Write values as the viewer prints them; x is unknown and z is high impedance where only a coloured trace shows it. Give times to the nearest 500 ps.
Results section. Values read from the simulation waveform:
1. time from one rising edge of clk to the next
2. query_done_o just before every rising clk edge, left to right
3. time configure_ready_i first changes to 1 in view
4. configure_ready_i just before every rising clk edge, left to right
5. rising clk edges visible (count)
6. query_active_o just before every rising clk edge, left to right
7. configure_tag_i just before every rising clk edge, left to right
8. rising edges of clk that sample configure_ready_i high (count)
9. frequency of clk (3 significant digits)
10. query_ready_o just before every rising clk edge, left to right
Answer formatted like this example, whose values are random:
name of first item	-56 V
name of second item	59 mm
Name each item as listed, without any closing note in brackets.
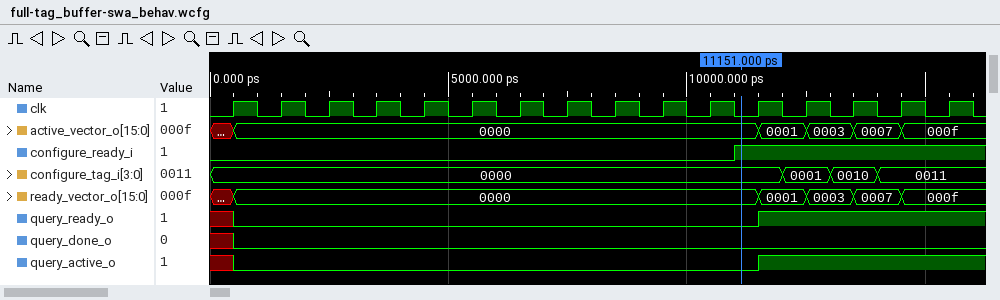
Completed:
time from one rising edge of clk to the next	1000 ps
query_done_o just before every rising clk edge, left to right	x 0 0 0 0 0 0 0 0 0 0 0 0 0 0 0
time configure_ready_i first changes to 1 in view	11000 ps
configure_ready_i just before every rising clk edge, left to right	0 0 0 0 0 0 0 0 0 0 0 1 1 1 1 1
rising clk edges visible	16
query_active_o just before every rising clk edge, left to right	x 0 0 0 0 0 0 0 0 0 0 0 1 1 1 1
configure_tag_i just before every rising clk edge, left to right	0000, 0000, 0000, 0000, 0000, 0000, 0000, 0000, 0000, 0000, 0000, 0000, 0001, 0010, 0011, 0011
rising edges of clk that sample configure_ready_i high	5
frequency of clk	1.00 GHz
query_ready_o just before every rising clk edge, left to right	x 0 0 0 0 0 0 0 0 0 0 0 1 1 1 1
